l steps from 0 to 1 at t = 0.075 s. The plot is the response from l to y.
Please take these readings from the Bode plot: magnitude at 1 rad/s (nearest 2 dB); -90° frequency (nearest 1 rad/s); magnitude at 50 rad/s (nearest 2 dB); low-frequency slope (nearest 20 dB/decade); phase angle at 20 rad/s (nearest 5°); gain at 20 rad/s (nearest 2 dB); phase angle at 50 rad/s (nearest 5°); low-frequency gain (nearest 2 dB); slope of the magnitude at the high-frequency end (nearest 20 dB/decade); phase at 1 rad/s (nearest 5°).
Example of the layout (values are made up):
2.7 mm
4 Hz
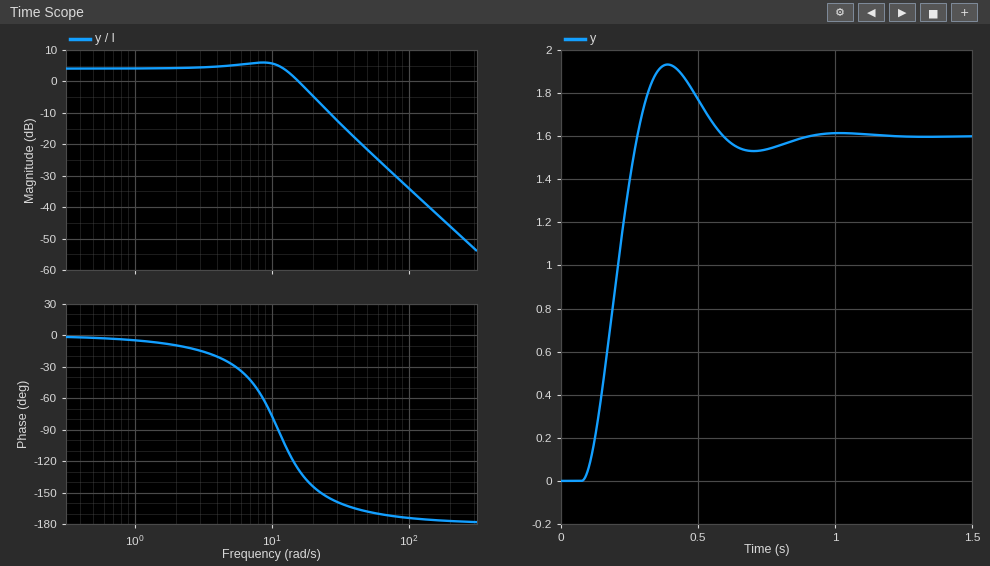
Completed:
4 dB
11 rad/s
-22 dB
0 dB/decade
-145°
-4 dB
-170°
4 dB
-40 dB/decade
-5°
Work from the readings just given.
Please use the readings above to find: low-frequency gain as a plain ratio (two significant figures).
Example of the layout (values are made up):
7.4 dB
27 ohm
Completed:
1.6
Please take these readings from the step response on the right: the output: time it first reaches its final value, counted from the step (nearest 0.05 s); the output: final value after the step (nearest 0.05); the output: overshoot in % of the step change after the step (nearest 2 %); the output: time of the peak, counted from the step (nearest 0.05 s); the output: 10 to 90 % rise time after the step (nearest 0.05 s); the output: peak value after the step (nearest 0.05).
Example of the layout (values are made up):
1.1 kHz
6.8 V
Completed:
0.20 s
1.60
20 %
0.30 s
0.15 s
1.95
